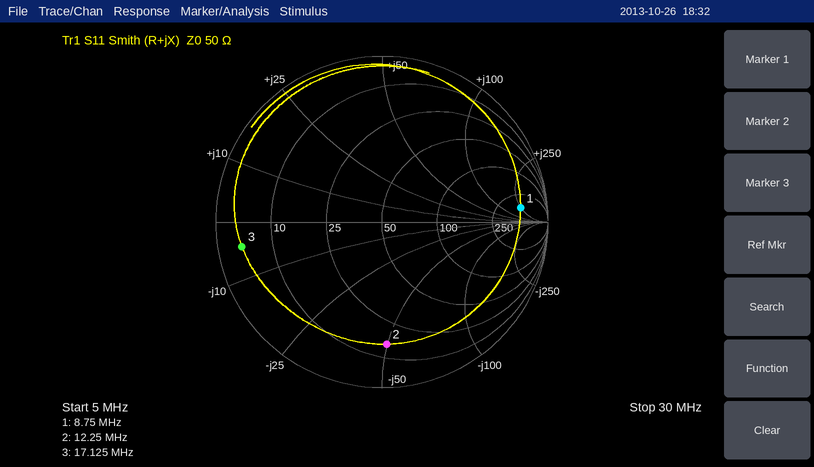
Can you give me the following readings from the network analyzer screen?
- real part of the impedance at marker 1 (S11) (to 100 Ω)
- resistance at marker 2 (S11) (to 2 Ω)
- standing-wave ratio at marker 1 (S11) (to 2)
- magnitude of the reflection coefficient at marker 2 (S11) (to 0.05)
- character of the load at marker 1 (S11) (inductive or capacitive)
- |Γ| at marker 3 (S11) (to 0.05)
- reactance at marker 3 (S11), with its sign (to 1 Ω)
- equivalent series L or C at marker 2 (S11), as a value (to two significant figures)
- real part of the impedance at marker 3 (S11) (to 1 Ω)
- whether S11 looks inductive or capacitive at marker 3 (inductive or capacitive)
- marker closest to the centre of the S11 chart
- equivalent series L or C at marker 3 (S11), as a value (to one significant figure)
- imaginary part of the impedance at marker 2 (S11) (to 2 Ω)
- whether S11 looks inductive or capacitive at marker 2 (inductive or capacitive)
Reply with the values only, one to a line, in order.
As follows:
400 Ω
16 Ω
12
0.75
inductive
0.85
-4 Ω
260 pF
4 Ω
capacitive
marker 2
2 nF
-50 Ω
capacitive
